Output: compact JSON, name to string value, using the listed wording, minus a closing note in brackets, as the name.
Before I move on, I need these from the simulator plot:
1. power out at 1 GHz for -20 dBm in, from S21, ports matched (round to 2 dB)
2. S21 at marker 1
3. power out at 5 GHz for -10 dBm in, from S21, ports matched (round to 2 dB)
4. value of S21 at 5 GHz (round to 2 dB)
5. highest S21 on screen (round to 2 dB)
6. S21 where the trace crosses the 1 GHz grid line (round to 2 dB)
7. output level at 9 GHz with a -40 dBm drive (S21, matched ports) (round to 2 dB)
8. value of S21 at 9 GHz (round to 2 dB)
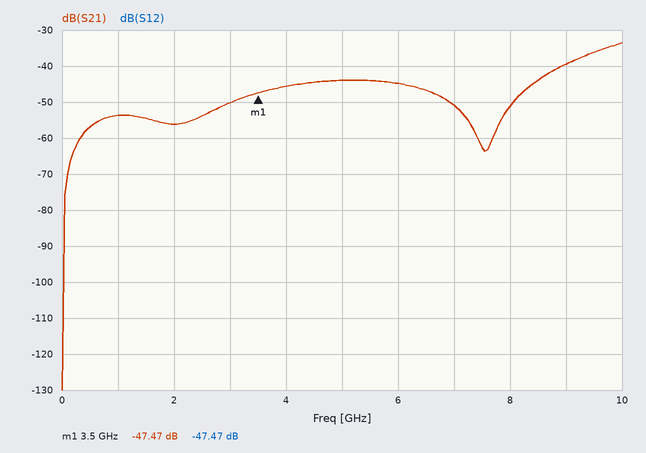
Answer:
{"power out at 1 GHz for -20 dBm in, from S21, ports matched": "-74 dBm", "S21 at marker 1": "-47.47 dB", "power out at 5 GHz for -10 dBm in, from S21, ports matched": "-54 dBm", "value of S21 at 5 GHz": "-44 dB", "highest S21 on screen": "-34 dB", "S21 where the trace crosses the 1 GHz grid line": "-54 dB", "output level at 9 GHz with a -40 dBm drive (S21, matched ports)": "-80 dBm", "value of S21 at 9 GHz": "-40 dB"}
